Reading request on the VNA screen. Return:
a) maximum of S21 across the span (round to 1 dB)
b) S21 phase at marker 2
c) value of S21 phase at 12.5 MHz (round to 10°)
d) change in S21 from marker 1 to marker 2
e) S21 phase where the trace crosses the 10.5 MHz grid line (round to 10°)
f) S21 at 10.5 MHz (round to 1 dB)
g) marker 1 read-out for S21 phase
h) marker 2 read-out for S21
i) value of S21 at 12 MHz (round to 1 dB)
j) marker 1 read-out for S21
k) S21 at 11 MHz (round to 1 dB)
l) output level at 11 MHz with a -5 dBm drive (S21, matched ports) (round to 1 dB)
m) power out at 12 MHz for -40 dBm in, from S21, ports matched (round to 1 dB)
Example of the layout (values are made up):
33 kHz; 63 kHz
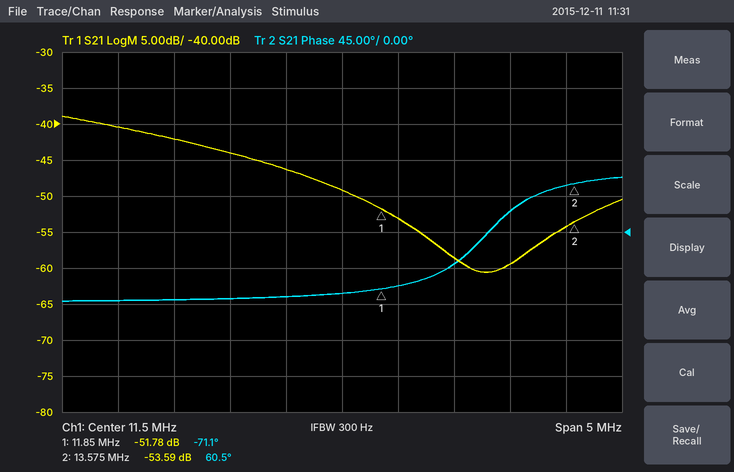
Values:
-39 dB; 60.5°; -40°; -1.81 dB; -80°; -44 dB; -71.1°; -53.59 dB; -53 dB; -51.78 dB; -46 dB; -51 dBm; -93 dBm
